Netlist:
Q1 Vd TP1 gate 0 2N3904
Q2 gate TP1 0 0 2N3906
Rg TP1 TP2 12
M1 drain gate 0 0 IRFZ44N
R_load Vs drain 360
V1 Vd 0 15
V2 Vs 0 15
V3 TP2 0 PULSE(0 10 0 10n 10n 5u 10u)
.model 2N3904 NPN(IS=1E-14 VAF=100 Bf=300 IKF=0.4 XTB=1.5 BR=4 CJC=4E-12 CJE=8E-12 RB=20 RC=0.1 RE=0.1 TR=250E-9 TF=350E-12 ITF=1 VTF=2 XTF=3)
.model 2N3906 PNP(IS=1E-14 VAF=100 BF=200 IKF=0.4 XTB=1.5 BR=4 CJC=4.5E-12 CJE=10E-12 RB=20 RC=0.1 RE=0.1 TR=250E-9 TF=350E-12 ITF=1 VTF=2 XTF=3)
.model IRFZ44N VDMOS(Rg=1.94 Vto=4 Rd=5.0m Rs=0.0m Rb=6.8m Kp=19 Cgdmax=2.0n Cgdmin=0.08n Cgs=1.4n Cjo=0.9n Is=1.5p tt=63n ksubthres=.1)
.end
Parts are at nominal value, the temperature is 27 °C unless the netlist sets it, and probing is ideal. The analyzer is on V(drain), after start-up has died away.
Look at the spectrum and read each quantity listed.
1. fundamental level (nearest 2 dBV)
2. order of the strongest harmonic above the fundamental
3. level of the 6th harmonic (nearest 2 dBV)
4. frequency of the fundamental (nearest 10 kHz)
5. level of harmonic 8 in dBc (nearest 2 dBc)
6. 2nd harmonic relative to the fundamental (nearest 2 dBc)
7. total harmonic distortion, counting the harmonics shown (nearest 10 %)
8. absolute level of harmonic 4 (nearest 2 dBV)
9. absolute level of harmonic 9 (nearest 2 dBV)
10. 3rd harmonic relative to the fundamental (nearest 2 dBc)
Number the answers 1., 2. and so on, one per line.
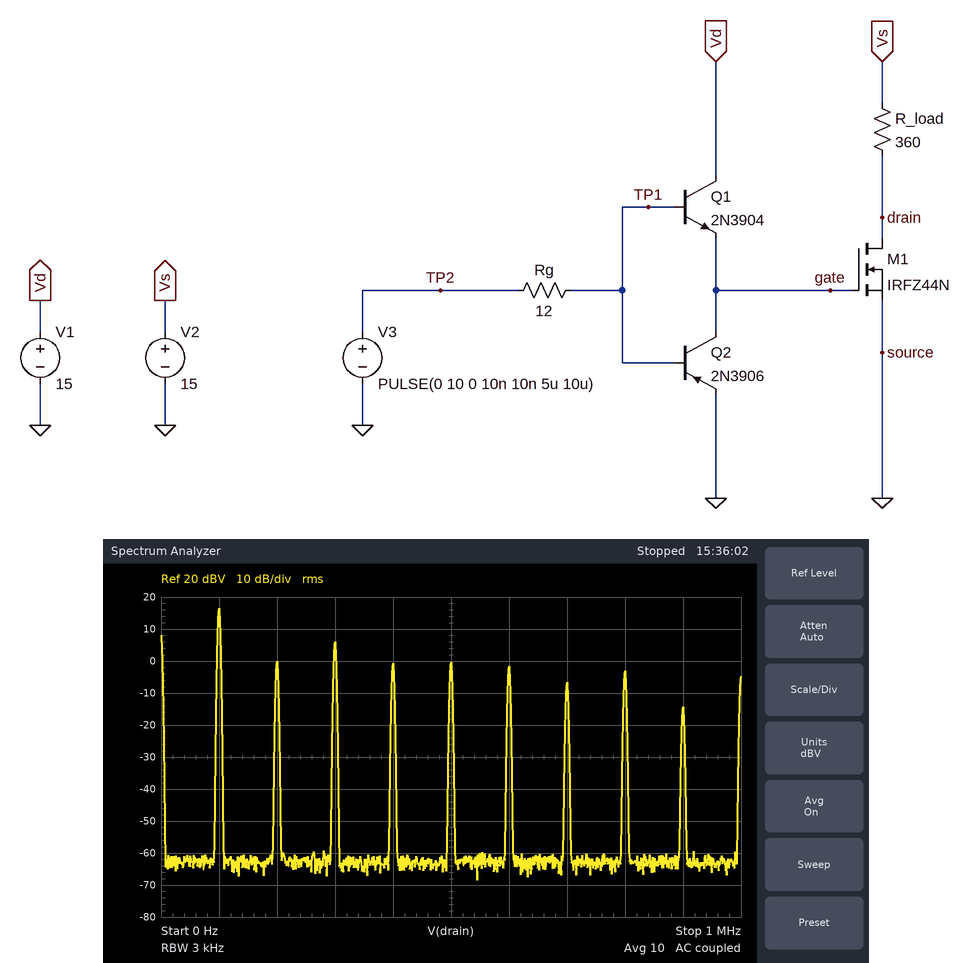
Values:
1. 16 dBV
2. 3
3. -2 dBV
4. 100 kHz
5. -20 dBc
6. -16 dBc
7. 40 %
8. 0 dBV
9. -14 dBV
10. -10 dBc
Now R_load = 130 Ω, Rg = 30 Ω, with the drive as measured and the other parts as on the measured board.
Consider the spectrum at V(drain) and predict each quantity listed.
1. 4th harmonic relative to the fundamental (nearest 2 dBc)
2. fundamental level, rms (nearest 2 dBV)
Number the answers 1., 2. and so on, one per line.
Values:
1. -22 dBc
2. 16 dBV
